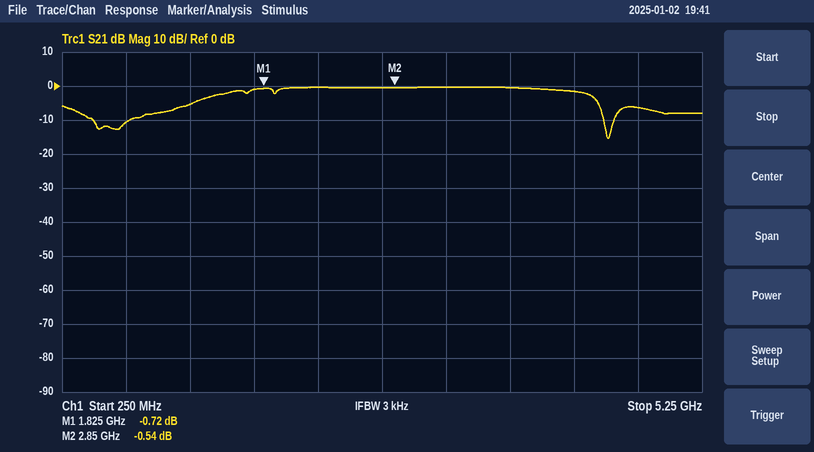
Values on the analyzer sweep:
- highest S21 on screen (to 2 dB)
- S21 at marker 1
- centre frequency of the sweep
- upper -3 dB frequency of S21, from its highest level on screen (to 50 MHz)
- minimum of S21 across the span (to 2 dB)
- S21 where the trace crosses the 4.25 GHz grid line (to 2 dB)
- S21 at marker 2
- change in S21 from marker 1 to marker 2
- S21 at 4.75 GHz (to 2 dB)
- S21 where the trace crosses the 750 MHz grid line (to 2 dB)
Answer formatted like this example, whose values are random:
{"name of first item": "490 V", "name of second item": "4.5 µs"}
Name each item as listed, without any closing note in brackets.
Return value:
{"highest S21 on screen": "0 dB", "S21 at marker 1": "-0.72 dB", "centre frequency of the sweep": "2.75 GHz", "upper -3 dB frequency of S21, from its highest level on screen": "4.40 GHz", "minimum of S21 across the span": "-16 dB", "S21 where the trace crosses the 4.25 GHz grid line": "-2 dB", "S21 at marker 2": "-0.54 dB", "change in S21 from marker 1 to marker 2": "0.18 dB", "S21 at 4.75 GHz": "-6 dB", "S21 where the trace crosses the 750 MHz grid line": "-10 dB"}
